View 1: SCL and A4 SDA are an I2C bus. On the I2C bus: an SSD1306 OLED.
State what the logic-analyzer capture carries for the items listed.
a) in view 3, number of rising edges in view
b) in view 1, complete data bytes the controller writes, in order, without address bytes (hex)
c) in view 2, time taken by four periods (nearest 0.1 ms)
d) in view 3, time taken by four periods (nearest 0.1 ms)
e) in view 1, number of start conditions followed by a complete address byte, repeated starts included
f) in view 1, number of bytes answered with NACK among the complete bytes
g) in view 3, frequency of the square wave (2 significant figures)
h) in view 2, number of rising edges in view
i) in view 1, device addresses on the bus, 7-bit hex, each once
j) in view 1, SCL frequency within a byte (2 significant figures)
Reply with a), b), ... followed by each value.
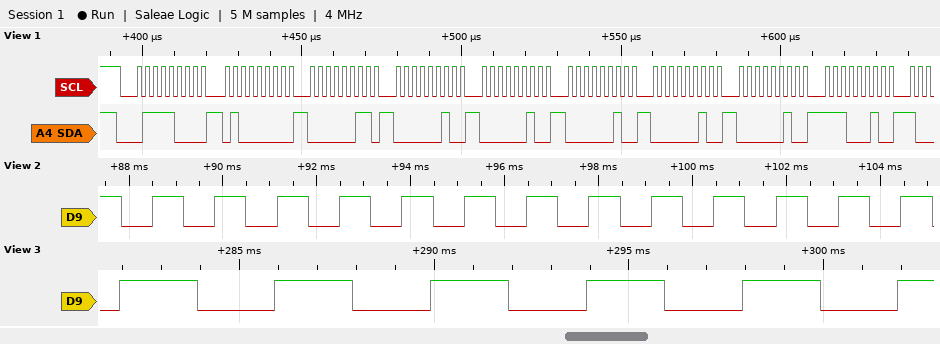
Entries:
a) 6
b) 40 03 02 02 02 02 02 E2
c) 5.3 ms
d) 16.0 ms
e) 1
f) 0
g) 250 Hz
h) 13
i) 0x3C
j) 400 kHz
